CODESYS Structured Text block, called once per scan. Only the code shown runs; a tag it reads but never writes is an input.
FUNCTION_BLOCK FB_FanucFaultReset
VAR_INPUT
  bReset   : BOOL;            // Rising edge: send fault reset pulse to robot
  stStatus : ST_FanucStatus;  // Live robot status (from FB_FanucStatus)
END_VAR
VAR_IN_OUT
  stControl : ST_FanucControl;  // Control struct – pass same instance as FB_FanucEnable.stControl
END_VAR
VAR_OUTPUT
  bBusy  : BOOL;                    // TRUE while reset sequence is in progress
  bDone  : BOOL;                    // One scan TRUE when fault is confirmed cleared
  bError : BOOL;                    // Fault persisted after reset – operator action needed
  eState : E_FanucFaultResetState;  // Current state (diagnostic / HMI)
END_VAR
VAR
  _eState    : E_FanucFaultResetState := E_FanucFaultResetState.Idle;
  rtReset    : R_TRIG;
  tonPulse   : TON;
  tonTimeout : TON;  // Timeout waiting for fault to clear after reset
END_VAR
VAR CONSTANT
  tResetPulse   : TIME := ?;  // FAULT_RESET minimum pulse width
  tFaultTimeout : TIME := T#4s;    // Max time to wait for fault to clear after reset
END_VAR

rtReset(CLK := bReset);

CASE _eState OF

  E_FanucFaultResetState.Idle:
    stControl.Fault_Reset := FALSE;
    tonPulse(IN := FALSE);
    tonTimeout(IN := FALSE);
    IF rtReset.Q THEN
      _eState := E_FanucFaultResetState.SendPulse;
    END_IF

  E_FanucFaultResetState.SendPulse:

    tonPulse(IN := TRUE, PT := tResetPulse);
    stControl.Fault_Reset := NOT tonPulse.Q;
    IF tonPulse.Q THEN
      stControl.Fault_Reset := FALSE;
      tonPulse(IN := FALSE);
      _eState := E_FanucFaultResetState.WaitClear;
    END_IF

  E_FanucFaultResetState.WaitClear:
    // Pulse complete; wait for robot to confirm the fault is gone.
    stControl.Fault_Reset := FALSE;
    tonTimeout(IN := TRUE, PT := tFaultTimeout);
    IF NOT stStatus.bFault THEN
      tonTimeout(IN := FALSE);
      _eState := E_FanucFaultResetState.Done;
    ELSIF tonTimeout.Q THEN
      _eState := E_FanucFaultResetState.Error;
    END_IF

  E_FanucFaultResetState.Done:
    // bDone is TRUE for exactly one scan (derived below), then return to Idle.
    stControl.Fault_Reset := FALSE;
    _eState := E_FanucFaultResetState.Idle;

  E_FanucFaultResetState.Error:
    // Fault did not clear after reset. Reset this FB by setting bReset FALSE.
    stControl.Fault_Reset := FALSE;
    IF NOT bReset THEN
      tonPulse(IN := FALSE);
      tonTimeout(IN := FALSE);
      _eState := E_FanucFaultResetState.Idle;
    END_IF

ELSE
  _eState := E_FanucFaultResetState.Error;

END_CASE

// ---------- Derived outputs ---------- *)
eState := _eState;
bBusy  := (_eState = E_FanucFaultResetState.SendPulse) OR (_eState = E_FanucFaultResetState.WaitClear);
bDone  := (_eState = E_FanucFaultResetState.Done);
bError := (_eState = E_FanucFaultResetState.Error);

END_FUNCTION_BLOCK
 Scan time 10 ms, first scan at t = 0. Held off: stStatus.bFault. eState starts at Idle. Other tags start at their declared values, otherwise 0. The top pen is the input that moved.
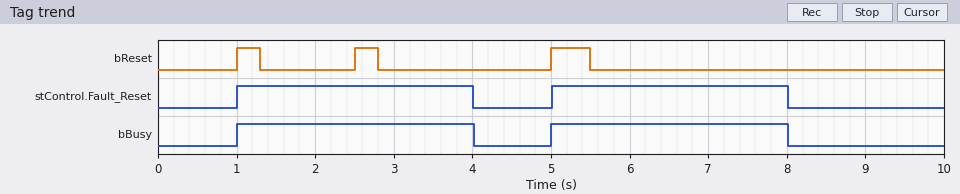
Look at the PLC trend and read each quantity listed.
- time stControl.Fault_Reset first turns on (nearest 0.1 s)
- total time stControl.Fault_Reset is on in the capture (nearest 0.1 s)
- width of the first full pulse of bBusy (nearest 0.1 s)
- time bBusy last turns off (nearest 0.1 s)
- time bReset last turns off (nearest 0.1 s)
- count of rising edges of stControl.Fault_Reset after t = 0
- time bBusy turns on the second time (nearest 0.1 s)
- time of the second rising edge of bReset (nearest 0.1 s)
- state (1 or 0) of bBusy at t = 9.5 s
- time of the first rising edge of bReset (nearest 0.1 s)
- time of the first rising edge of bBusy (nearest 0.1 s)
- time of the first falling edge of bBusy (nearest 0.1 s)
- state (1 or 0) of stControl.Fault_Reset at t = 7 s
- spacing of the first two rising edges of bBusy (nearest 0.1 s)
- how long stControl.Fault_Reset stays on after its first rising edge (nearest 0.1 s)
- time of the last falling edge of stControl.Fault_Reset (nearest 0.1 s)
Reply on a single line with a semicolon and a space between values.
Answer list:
1.0 s; 6.0 s; 3.0 s; 8.0 s; 5.5 s; 2; 5.0 s; 2.5 s; 0; 1.0 s; 1.0 s; 4.0 s; 1; 4.0 s; 3.0 s; 8.0 s
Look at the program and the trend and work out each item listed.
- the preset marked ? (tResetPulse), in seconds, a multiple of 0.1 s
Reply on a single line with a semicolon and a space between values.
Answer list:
3.0 s
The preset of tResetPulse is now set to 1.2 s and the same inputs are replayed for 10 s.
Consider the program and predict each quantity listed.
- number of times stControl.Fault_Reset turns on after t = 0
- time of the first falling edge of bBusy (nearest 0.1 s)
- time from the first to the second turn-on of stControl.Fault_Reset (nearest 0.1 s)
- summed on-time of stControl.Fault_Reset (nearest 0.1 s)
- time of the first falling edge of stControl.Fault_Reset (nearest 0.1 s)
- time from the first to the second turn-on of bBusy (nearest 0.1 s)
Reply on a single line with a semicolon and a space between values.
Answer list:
3; 2.2 s; 1.5 s; 3.6 s; 2.2 s; 1.5 s
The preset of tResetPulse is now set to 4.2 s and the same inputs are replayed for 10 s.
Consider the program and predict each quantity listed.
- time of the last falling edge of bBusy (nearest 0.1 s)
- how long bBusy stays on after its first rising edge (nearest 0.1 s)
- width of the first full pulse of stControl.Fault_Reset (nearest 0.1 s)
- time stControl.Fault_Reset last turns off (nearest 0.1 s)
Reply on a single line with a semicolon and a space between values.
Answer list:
5.2 s; 4.2 s; 4.2 s; 5.2 s
